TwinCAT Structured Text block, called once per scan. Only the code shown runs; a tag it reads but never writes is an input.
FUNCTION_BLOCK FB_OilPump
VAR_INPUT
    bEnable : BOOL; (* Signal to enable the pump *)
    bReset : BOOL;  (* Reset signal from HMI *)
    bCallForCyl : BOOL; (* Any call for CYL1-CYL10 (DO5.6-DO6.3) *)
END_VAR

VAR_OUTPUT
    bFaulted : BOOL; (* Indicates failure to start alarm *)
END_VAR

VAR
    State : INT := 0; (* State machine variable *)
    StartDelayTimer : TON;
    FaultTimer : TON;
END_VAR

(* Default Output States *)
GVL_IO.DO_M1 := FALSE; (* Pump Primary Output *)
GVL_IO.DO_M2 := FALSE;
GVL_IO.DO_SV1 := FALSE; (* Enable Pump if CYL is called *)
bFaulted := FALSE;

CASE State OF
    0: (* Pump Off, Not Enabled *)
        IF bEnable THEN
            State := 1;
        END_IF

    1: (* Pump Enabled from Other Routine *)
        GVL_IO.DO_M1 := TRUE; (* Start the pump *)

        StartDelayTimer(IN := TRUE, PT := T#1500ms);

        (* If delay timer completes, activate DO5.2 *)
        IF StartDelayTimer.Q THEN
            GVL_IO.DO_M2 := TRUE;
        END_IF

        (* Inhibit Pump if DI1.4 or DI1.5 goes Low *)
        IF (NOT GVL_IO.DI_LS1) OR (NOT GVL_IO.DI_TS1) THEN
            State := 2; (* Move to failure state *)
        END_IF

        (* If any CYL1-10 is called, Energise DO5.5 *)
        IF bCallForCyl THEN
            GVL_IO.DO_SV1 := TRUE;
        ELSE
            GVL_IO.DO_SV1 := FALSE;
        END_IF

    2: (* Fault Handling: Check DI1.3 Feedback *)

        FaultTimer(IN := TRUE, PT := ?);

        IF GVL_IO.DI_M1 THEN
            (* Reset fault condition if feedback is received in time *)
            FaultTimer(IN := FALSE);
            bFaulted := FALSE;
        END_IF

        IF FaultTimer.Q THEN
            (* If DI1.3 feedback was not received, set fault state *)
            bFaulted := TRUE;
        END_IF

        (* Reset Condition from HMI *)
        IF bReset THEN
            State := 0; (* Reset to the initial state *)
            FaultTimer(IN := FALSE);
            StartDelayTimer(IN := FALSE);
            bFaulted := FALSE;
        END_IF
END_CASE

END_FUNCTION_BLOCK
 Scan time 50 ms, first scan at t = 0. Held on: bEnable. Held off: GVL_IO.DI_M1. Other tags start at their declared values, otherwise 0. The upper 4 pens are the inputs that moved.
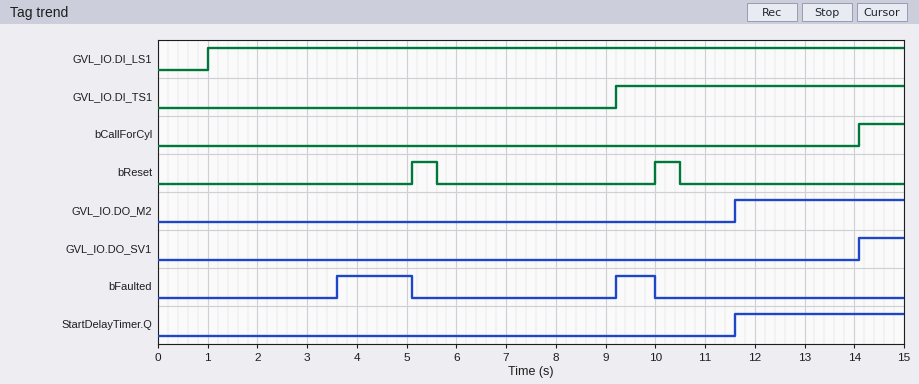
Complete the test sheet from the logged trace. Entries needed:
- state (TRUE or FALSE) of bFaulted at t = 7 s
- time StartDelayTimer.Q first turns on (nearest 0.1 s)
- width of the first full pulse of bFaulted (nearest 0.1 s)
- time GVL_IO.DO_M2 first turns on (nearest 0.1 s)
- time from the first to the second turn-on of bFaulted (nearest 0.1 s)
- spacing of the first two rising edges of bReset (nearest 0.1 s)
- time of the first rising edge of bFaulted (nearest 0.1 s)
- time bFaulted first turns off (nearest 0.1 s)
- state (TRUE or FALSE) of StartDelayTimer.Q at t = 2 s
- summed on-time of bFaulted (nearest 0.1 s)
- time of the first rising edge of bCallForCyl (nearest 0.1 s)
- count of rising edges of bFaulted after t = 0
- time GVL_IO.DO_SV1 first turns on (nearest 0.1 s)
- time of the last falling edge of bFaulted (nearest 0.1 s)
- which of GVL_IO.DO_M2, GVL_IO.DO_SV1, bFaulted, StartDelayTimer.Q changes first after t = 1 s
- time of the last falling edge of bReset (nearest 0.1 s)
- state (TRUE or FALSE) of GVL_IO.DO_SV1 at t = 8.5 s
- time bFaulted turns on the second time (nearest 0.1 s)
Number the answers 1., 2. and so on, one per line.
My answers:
1. FALSE
2. 11.6 s
3. 1.5 s
4. 11.6 s
5. 5.6 s
6. 4.9 s
7. 3.6 s
8. 5.1 s
9. FALSE
10. 2.3 s
11. 14.1 s
12. 2
13. 14.1 s
14. 10.0 s
15. bFaulted
16. 10.5 s
17. FALSE
18. 9.2 s
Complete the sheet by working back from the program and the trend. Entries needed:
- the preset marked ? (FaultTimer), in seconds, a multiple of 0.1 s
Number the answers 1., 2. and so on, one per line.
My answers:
1. 3.5 s
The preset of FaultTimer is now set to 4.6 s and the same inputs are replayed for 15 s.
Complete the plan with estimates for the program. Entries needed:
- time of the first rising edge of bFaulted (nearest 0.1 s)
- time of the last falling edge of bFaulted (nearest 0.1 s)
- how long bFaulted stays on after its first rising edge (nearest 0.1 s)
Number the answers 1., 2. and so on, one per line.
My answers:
1. 4.7 s
2. 5.1 s
3. 0.4 s
